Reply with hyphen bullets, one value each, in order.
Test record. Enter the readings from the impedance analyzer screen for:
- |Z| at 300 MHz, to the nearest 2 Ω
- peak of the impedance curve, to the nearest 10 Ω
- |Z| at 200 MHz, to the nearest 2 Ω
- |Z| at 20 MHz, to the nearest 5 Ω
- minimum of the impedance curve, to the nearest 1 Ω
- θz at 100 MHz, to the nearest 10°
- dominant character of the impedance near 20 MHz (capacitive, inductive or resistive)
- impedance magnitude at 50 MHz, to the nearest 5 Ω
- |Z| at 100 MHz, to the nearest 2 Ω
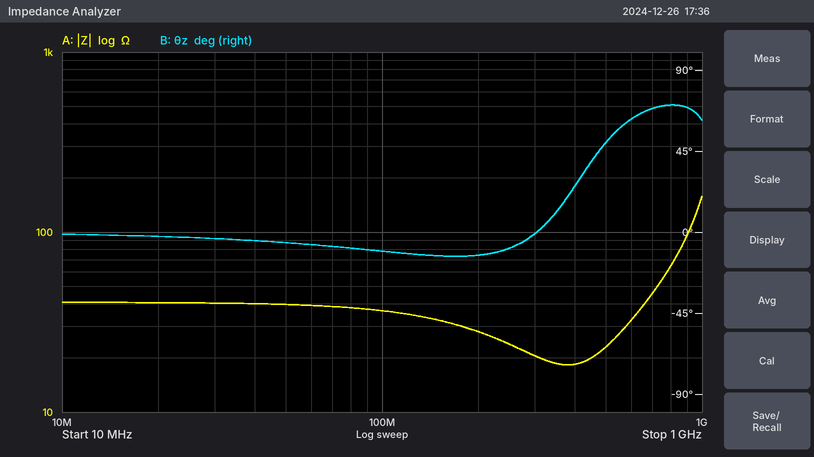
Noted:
- 20 Ω
- 160 Ω
- 28 Ω
- 40 Ω
- 18 Ω
- -10°
- resistive
- 40 Ω
- 36 Ω
